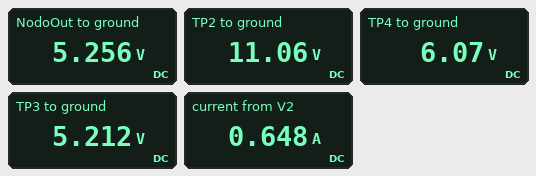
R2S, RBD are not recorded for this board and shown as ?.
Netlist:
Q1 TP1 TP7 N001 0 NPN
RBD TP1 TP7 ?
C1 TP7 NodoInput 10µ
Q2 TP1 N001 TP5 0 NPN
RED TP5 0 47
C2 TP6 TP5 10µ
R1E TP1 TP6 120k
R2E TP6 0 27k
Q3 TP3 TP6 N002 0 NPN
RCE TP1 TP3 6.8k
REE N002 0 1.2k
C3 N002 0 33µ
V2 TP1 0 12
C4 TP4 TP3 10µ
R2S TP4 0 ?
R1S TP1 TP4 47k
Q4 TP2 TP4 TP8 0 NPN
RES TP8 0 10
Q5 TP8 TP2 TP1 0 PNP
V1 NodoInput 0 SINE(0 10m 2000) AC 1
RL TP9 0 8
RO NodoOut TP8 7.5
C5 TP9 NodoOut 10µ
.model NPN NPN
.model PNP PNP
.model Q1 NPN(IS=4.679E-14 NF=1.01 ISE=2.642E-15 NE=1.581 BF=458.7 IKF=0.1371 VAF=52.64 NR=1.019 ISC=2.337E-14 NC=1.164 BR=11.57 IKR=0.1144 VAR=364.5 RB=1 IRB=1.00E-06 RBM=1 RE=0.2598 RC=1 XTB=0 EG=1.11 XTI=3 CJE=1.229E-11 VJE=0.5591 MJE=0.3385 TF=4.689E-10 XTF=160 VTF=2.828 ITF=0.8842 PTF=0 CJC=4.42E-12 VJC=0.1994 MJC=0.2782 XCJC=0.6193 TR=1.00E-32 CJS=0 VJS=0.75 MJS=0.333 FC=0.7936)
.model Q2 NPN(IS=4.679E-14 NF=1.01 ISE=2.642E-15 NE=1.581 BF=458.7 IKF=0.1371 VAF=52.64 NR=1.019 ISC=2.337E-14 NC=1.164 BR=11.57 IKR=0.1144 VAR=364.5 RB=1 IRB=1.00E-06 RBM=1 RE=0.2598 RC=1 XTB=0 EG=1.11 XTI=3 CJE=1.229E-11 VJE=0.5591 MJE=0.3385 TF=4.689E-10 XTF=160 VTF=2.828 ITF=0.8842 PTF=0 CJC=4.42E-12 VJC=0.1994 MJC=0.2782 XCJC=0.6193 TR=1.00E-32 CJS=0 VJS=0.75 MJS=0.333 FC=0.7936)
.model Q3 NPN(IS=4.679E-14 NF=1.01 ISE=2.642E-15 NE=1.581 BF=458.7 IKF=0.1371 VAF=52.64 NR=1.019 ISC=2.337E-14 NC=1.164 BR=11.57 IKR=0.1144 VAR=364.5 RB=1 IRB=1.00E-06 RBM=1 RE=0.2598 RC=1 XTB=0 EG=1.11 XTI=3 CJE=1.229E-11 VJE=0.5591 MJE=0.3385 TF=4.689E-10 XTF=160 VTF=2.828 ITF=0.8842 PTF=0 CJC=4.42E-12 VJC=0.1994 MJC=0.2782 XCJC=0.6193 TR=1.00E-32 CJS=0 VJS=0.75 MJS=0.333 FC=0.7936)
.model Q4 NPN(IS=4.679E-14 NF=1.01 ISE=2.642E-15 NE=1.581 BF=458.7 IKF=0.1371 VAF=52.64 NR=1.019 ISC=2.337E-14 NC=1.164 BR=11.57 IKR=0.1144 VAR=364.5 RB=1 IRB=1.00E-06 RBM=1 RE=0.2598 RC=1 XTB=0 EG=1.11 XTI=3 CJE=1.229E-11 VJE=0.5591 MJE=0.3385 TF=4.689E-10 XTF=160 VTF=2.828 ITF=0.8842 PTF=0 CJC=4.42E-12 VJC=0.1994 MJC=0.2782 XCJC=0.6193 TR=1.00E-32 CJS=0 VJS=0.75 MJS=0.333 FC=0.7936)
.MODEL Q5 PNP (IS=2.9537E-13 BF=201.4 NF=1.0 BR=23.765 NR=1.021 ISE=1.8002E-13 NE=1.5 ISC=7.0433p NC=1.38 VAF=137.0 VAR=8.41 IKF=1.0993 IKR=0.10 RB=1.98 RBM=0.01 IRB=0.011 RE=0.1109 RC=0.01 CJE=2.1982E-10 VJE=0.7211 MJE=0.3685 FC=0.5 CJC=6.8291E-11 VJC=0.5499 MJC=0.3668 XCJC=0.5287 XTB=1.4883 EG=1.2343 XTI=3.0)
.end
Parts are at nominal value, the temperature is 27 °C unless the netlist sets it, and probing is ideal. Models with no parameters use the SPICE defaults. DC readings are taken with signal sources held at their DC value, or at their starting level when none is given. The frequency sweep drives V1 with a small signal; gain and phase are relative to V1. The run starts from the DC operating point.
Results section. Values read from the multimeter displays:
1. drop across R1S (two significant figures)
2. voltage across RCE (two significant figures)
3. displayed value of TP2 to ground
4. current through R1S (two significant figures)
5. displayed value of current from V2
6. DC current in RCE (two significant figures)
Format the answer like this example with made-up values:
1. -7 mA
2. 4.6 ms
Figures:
1. 5.9 V
2. 6.8 V
3. 11.06 V
4. 130 µA
5. 0.648 A
6. 1.0 mA
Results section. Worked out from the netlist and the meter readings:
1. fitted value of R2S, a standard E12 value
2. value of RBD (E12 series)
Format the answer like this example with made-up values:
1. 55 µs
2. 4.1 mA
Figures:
1. 82 kΩ
2. 390 kΩ
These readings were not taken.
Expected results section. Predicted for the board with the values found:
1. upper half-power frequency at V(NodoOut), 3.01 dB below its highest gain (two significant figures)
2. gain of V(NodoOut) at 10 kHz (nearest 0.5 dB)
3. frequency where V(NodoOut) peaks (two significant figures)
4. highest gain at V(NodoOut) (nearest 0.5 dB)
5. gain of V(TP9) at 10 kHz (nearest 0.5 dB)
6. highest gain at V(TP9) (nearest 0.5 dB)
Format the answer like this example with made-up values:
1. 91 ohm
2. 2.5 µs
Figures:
1. 2.3 kHz
2. 40.0 dB
3. 490 Hz
4. 44.5 dB
5. 40.0 dB
6. 40.0 dB
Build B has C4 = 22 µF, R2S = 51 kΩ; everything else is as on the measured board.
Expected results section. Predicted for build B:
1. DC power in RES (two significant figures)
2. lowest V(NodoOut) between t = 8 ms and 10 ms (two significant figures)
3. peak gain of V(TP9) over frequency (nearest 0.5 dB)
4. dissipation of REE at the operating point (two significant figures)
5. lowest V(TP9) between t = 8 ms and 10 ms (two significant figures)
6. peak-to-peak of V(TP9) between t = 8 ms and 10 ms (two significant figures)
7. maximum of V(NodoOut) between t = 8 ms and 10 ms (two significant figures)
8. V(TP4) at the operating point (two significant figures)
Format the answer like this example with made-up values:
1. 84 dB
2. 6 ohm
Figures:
1. 1.9 W
2. 3.1 V
3. 39.5 dB
4. 1.2 mW
5. -910 mV
6. 1.7 V
7. 5.5 V
8. 5.2 V
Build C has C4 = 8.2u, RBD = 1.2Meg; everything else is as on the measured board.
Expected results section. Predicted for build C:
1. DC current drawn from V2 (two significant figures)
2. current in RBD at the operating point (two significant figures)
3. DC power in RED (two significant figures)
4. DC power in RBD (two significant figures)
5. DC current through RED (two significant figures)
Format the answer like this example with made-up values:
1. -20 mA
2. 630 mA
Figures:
1. 590 mA
2. 6.2 µA
3. 190 mW
4. 46 µW
5. 63 mA
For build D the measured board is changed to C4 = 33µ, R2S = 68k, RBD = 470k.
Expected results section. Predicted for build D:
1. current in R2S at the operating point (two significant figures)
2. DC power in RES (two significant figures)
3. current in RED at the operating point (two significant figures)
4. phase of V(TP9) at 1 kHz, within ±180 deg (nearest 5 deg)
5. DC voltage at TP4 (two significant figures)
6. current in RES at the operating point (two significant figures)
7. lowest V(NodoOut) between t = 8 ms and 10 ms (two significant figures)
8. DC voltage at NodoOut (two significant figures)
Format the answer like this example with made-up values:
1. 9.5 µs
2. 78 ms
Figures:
1. 84 µA
2. 2.4 W
3. 110 mA
4. -125 deg
5. 5.7 V
6. 490 mA
7. 3.6 V
8. 4.9 V
